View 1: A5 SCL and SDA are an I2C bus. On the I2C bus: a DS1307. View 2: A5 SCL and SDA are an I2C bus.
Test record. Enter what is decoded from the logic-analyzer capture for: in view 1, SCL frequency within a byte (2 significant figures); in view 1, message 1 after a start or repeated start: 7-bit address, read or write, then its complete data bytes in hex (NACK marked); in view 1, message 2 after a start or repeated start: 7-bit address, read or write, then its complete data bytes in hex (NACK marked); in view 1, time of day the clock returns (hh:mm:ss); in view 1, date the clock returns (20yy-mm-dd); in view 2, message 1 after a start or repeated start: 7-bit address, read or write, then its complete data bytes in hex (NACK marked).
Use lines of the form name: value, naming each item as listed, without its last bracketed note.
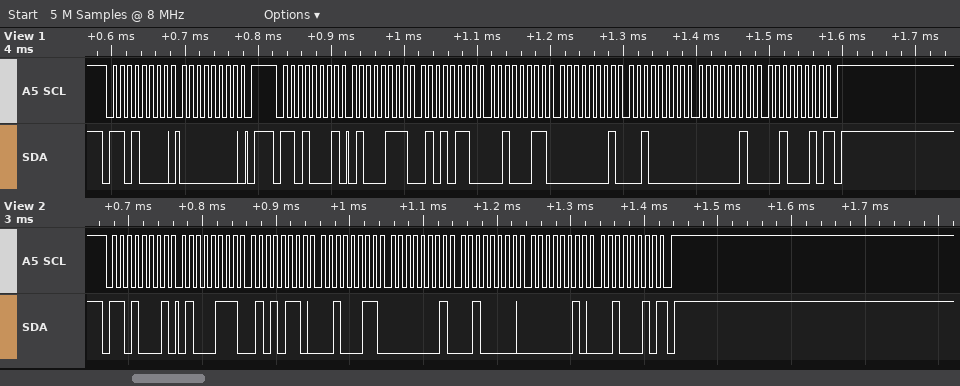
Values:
in view 1, SCL frequency within a byte: 100 kHz
in view 1, message 1 after a start or repeated start: 7-bit address, read or write, then its complete data bytes in hex: 0x68 write: 00
in view 1, message 2 after a start or repeated start: 7-bit address, read or write, then its complete data bytes in hex: 0x68 read: 47 56 23 01 20 02 22 NACK
in view 1, time of day the clock returns: 23:56:47
in view 1, date the clock returns: 2022-02-20
in view 2, message 1 after a start or repeated start: 7-bit address, read or write, then its complete data bytes in hex: 0x68 read: 47 56 23 01 20 02 22 NACK
